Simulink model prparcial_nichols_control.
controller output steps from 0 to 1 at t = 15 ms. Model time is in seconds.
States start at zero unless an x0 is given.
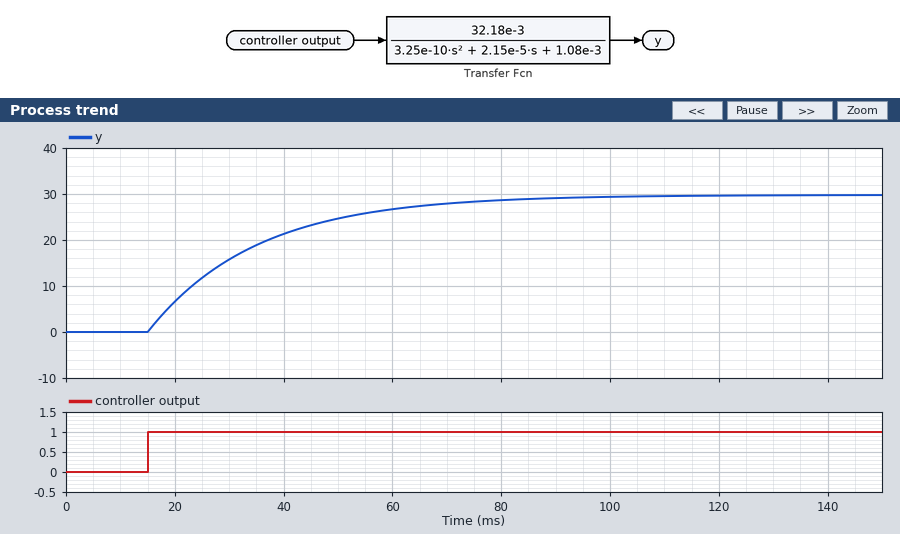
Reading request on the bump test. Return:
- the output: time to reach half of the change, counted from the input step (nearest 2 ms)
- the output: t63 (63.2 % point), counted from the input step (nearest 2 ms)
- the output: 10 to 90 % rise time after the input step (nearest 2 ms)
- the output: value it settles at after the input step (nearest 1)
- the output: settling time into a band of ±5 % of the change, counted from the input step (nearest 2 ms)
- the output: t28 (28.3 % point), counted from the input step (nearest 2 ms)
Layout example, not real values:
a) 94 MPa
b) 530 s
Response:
a) 14 ms
b) 20 ms
c) 44 ms
d) 30
e) 60 ms
f) 6 ms
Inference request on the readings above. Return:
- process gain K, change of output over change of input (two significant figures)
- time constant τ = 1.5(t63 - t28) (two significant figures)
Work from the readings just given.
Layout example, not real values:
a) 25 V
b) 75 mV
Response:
a) 30
b) 21 ms
